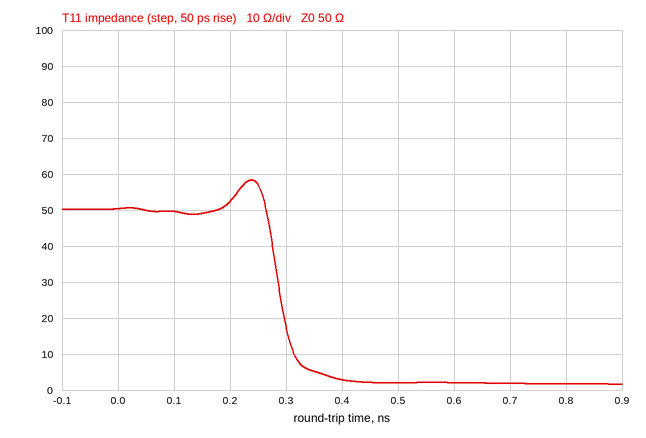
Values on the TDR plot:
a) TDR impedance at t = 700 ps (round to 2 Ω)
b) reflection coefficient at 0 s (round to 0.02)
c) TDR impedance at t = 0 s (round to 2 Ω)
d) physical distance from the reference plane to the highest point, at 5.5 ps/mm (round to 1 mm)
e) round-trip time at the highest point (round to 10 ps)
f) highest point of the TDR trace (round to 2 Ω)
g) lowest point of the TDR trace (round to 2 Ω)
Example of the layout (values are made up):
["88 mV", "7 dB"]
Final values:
["2 Ω", "0.00", "50 Ω", "22 mm", "240 ps", "58 Ω", "2 Ω"]
